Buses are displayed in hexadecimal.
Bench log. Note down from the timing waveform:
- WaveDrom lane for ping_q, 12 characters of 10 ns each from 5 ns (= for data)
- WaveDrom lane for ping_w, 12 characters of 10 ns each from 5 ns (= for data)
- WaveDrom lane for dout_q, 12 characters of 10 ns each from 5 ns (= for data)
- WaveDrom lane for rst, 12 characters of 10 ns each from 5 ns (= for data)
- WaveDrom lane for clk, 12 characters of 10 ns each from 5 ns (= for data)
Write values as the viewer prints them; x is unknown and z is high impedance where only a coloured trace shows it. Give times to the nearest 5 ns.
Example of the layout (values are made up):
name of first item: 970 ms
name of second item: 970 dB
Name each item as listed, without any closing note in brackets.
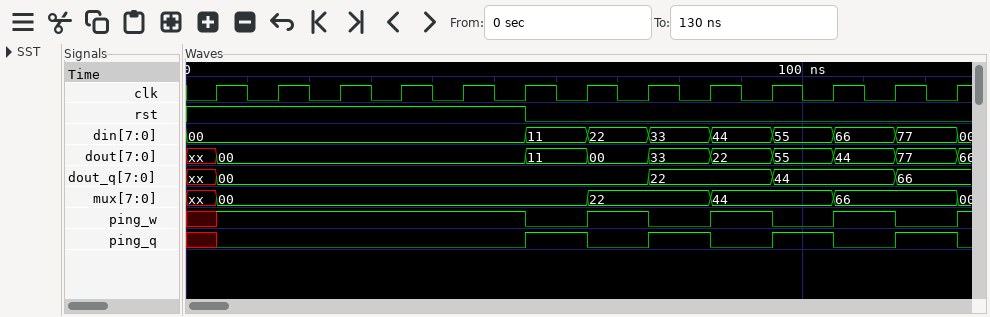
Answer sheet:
WaveDrom lane for ping_q, 12 characters of 10 ns each from 5 ns: {name: 'ping_q', wave: '0....1010101'}
WaveDrom lane for ping_w, 12 characters of 10 ns each from 5 ns: {name: 'ping_w', wave: '1....0101010'}
WaveDrom lane for dout_q, 12 characters of 10 ns each from 5 ns: {name: 'dout_q', wave: '=......=.=.=', data: '00 22 44 66'}
WaveDrom lane for rst, 12 characters of 10 ns each from 5 ns: {name: 'rst', wave: '1....0......'}
WaveDrom lane for clk, 12 characters of 10 ns each from 5 ns: {name: 'clk', wave: 'p...........'}
